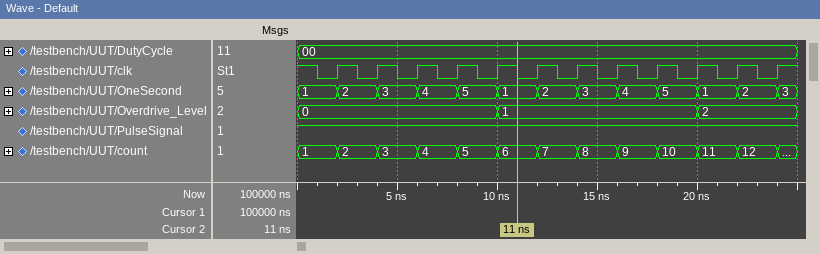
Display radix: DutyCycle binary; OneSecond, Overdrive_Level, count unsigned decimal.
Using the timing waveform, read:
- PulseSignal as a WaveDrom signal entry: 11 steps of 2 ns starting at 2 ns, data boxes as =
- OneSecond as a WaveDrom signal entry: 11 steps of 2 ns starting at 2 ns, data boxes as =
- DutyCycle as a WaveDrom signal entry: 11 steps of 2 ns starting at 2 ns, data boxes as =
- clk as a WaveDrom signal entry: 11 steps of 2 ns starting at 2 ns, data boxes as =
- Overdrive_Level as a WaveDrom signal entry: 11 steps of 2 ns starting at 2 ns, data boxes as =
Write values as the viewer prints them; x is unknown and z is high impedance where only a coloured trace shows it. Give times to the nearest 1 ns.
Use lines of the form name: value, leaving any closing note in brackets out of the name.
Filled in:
PulseSignal as a WaveDrom signal entry: 11 steps of 2 ns starting at 2 ns, data boxes as =: {name: 'PulseSignal', wave: '1..........'}
OneSecond as a WaveDrom signal entry: 11 steps of 2 ns starting at 2 ns, data boxes as =: {name: 'OneSecond', wave: '===========', data: '2 3 4 5 1 2 3 4 5 1 2'}
DutyCycle as a WaveDrom signal entry: 11 steps of 2 ns starting at 2 ns, data boxes as =: {name: 'DutyCycle', wave: '=..........', data: '00'}
clk as a WaveDrom signal entry: 11 steps of 2 ns starting at 2 ns, data boxes as =: {name: 'clk', wave: 'p..........'}
Overdrive_Level as a WaveDrom signal entry: 11 steps of 2 ns starting at 2 ns, data boxes as =: {name: 'Overdrive_Level', wave: '=...=....=.', data: '0 1 2'}
